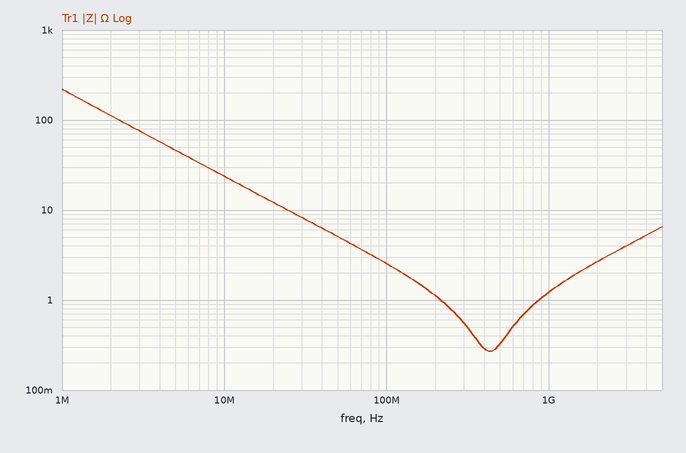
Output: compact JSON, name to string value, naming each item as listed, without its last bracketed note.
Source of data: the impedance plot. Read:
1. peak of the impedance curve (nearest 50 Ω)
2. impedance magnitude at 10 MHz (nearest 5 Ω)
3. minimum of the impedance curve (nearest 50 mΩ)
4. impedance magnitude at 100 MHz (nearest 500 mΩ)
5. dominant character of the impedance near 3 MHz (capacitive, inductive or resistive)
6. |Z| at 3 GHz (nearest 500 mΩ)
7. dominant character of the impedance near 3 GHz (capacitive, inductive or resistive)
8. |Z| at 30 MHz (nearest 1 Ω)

{"peak of the impedance curve": "200 Ω", "impedance magnitude at 10 MHz": "25 Ω", "minimum of the impedance curve": "250 mΩ", "impedance magnitude at 100 MHz": "2.5 Ω", "dominant character of the impedance near 3 MHz": "capacitive", "|Z| at 3 GHz": "4.0 Ω", "dominant character of the impedance near 3 GHz": "inductive", "|Z| at 30 MHz": "8 Ω"}
